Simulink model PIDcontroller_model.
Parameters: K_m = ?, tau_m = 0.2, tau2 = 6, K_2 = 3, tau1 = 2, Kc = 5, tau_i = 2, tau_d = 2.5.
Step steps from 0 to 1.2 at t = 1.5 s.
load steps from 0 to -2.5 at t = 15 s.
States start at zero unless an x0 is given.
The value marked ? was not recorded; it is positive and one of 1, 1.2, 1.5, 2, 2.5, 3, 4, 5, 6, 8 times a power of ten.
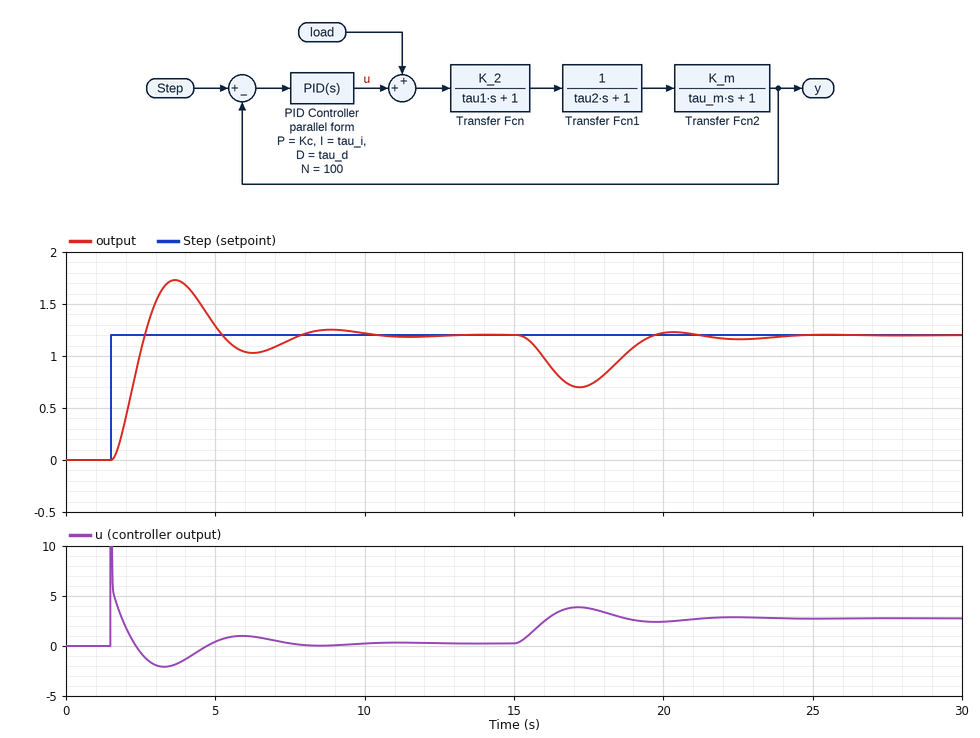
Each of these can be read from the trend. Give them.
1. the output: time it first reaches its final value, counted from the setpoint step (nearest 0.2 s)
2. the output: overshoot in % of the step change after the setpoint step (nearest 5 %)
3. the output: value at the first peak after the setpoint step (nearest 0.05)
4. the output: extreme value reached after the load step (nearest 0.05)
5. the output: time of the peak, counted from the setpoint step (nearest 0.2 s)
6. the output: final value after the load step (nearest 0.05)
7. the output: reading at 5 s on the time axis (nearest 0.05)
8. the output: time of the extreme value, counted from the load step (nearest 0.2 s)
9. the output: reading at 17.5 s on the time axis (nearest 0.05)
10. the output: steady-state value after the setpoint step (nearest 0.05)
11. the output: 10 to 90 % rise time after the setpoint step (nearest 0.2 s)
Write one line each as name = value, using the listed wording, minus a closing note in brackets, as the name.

the output: time it first reaches its final value, counted from the setpoint step = 1.2 s
the output: overshoot in % of the step change after the setpoint step = 45 %
the output: value at the first peak after the setpoint step = 1.75
the output: extreme value reached after the load step = 0.70
the output: time of the peak, counted from the setpoint step = 2.2 s
the output: final value after the load step = 1.20
the output: reading at 5 s on the time axis = 1.30
the output: time of the extreme value, counted from the load step = 2.2 s
the output: reading at 17.5 s on the time axis = 0.70
the output: steady-state value after the setpoint step = 1.20
the output: 10 to 90 % rise time after the setpoint step = 0.8 s
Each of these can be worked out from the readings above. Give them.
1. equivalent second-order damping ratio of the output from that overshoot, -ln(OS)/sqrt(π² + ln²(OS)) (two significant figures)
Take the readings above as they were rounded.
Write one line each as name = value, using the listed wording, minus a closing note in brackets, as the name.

equivalent second-order damping ratio of the output from that overshoot, -ln(OS)/sqrt(π² + ln²(OS)) = 0.25
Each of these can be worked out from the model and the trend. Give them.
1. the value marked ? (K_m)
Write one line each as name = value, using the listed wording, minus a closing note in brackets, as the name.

the value marked ? = 1.5
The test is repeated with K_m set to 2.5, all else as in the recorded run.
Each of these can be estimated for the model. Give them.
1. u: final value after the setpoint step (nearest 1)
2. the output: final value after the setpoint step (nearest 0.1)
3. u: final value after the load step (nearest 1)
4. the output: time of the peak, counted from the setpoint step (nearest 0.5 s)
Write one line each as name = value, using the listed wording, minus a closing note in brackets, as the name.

u: final value after the setpoint step = 0
the output: final value after the setpoint step = 1.2
u: final value after the load step = 3
the output: time of the peak, counted from the setpoint step = 1.5 s
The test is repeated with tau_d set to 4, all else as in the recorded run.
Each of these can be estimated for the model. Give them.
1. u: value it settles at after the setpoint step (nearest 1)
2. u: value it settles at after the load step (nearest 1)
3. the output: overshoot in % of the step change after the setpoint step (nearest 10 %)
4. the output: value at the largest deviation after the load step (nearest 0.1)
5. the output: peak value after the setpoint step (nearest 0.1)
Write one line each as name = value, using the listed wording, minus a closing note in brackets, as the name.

u: value it settles at after the setpoint step = 0
u: value it settles at after the load step = 3
the output: overshoot in % of the step change after the setpoint step = 30 %
the output: value at the largest deviation after the load step = 0.8
the output: peak value after the setpoint step = 1.5
